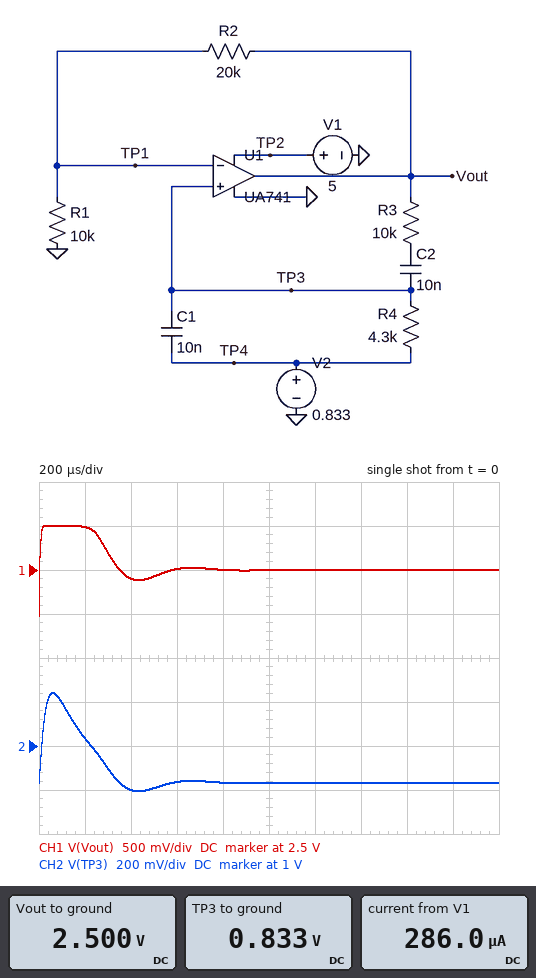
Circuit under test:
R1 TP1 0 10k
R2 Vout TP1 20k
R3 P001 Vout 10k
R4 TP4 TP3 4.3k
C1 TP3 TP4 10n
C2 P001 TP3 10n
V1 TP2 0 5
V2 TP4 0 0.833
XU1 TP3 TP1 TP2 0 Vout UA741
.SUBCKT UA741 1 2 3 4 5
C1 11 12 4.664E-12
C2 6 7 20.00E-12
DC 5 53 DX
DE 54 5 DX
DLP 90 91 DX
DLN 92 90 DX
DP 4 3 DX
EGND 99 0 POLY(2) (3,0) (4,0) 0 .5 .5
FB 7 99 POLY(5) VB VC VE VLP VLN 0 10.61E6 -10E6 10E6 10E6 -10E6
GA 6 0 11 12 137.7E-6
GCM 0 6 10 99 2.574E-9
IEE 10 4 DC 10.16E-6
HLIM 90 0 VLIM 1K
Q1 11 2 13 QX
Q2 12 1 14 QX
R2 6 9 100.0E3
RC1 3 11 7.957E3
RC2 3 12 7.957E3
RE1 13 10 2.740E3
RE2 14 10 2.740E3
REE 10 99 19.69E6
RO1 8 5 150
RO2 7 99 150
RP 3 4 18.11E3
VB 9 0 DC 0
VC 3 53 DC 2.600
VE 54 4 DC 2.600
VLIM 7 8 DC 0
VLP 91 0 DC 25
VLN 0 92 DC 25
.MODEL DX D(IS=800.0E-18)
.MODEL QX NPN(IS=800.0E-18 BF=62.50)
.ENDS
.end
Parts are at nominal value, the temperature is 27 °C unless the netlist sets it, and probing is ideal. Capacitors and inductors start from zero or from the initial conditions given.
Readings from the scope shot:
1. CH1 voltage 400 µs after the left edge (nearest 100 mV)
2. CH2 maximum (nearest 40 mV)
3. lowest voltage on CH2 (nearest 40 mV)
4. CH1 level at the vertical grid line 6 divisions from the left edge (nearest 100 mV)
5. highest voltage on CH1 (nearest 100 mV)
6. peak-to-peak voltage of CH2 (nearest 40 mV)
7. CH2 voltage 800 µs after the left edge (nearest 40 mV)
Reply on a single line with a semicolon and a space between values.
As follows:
2.4 V; 1.24 V; 800 mV; 2.5 V; 3.0 V; 440 mV; 840 mV
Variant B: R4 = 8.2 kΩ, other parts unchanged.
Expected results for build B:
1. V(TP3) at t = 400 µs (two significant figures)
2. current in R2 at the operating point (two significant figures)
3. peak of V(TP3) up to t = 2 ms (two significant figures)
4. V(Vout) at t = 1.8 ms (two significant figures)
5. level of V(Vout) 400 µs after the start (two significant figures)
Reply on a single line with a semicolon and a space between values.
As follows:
980 mV; 83 µA; 1.4 V; 2.4 V; 2.9 V
